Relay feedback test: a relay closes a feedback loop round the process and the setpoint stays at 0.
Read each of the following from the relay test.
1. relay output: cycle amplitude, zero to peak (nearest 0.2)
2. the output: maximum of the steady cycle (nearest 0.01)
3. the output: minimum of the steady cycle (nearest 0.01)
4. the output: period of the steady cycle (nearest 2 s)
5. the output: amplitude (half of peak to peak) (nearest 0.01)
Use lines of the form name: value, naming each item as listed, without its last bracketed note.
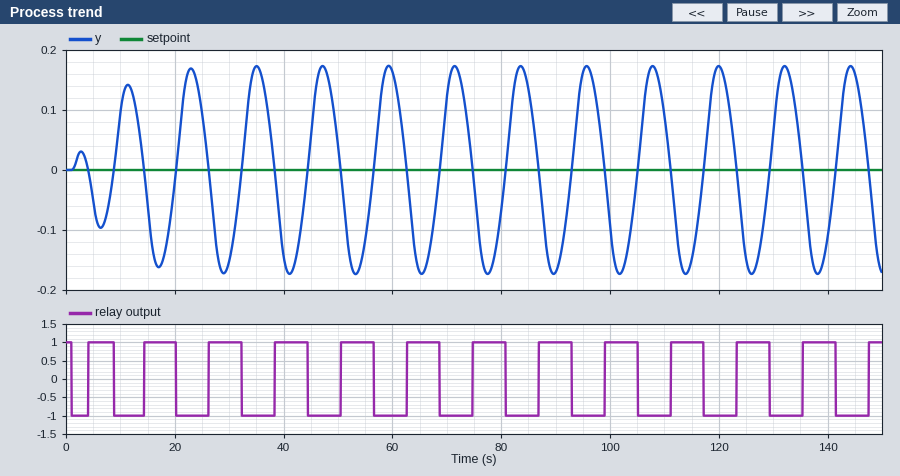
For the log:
relay output: cycle amplitude, zero to peak: 1.0
the output: maximum of the steady cycle: 0.17
the output: minimum of the steady cycle: -0.17
the output: period of the steady cycle: 12 s
the output: amplitude (half of peak to peak): 0.17
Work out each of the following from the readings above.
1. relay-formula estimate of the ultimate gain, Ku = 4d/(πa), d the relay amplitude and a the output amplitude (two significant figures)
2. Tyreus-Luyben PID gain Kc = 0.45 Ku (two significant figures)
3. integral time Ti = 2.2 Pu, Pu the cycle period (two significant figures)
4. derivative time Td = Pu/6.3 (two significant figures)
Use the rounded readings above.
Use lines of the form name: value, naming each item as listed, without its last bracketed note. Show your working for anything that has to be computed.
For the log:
relay-formula estimate of the ultimate gain, Ku = 4d/(πa), d the relay amplitude and a the output amplitude: 4 × 1 / (π × 0.17) = 7.5
Tyreus-Luyben PID gain Kc = 0.45 Ku: 0.45 × 7.5 = 3.4
integral time Ti = 2.2 Pu, Pu the cycle period: 2.2 × 12 = 26 s
derivative time Td = Pu/6.3: 12 / 6.3 = 1.9 s
